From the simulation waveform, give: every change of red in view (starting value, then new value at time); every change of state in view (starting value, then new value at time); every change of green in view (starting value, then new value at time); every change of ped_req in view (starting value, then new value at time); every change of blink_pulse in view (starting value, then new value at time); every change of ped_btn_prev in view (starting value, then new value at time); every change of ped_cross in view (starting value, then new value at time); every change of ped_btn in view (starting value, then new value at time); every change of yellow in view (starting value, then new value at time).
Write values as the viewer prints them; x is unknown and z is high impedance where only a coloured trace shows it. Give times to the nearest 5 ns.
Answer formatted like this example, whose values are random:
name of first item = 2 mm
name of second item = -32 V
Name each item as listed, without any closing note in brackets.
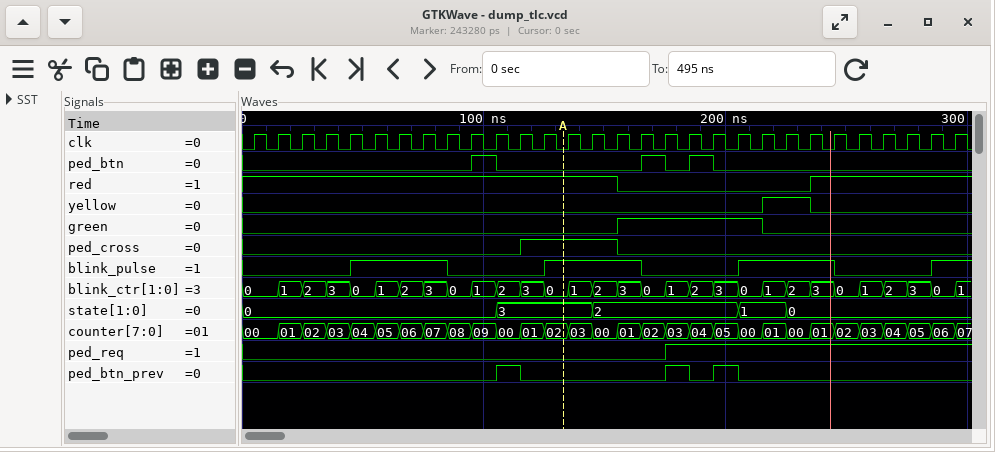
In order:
every change of red in view = 1, 0 at 155 ns, 1 at 235 ns
every change of state in view = 0, 3 at 105 ns, 2 at 145 ns, 1 at 205 ns, 0 at 225 ns
every change of green in view = 0, 1 at 155 ns, 0 at 215 ns
every change of ped_req in view = 0, 1 at 175 ns
every change of blink_pulse in view = 0, 1 at 45 ns, 0 at 85 ns, 1 at 125 ns, 0 at 165 ns, 1 at 205 ns, 0 at 245 ns, 1 at 285 ns
every change of ped_btn_prev in view = 0, 1 at 105 ns, 0 at 115 ns, 1 at 175 ns, 0 at 185 ns, 1 at 195 ns, 0 at 205 ns
every change of ped_cross in view = 0, 1 at 115 ns, 0 at 155 ns
every change of ped_btn in view = 0, 1 at 95 ns, 0 at 105 ns, 1 at 165 ns, 0 at 175 ns, 1 at 185 ns, 0 at 195 ns
every change of yellow in view = 0, 1 at 215 ns, 0 at 235 ns
